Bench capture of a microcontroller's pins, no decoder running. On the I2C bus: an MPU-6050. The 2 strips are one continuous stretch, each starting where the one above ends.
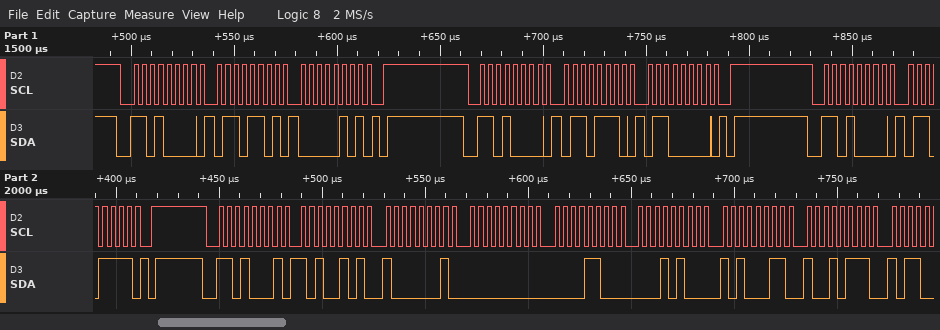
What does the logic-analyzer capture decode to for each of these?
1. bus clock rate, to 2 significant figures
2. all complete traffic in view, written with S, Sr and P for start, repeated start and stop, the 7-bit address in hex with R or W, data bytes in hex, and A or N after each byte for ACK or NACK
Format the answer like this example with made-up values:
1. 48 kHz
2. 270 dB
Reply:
1. 250 kHz
2. S 68W A 6D A 05 A P S 68W A 6E A 60 A P S 68W A 6F A P S 68R A A5 A 81 A 00 A 0C A 14 A A3 A 97 A
